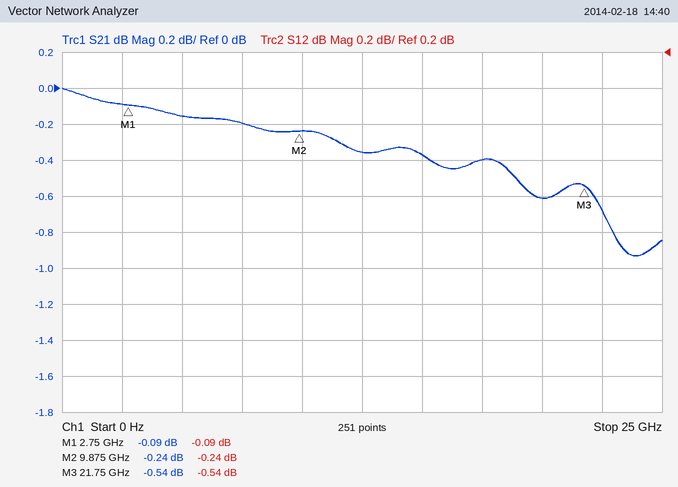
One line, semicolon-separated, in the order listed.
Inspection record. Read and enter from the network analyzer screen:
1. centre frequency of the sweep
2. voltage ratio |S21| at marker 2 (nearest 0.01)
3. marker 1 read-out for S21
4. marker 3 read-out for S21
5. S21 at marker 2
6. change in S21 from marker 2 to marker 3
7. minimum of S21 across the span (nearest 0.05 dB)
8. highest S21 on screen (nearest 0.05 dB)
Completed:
12.5 GHz; 0.97; -0.09 dB; -0.54 dB; -0.24 dB; -0.30 dB; -0.95 dB; 0.00 dB
